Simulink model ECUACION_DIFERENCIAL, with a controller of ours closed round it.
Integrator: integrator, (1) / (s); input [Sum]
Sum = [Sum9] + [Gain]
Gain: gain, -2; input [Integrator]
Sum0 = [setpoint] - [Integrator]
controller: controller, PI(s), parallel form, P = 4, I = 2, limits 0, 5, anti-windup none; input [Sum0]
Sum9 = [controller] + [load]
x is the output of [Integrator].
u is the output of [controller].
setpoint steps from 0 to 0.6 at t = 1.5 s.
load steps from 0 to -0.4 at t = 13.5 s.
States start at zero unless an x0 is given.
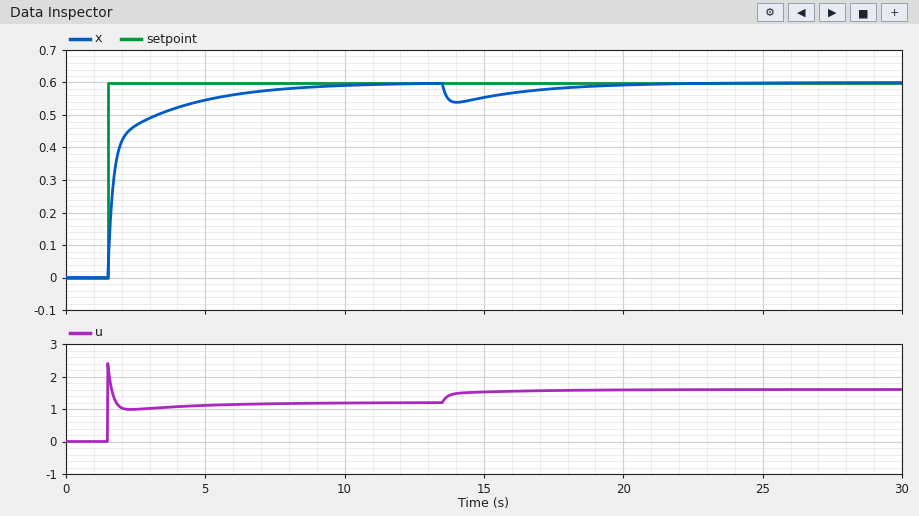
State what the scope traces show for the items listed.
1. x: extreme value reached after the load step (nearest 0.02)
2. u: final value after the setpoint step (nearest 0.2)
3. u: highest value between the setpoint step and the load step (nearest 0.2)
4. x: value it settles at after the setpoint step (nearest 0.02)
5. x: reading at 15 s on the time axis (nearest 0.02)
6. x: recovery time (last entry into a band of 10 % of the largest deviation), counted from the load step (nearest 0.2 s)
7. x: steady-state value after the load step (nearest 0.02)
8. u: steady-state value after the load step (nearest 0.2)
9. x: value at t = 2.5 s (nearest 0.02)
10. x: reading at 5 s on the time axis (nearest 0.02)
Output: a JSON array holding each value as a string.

["0.54", "1.2", "2.4", "0.60", "0.56", "7.4 s", "0.60", "1.6", "0.46", "0.54"]
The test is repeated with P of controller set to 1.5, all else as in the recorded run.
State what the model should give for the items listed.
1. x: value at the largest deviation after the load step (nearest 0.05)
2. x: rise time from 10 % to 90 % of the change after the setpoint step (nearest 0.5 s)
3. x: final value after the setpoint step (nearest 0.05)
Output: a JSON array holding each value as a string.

["0.50", "2.5 s", "0.60"]
